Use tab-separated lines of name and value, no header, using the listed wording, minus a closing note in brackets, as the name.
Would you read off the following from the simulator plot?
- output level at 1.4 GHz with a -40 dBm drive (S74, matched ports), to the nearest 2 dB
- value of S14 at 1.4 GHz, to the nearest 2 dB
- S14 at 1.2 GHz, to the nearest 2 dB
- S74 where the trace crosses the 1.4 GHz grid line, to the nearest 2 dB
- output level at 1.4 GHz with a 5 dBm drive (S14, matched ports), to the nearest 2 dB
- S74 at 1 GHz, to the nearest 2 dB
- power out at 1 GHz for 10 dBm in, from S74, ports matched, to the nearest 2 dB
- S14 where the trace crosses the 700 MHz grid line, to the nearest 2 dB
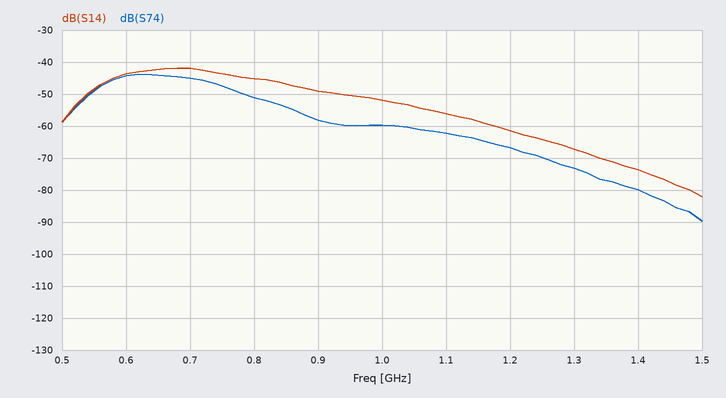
output level at 1.4 GHz with a -40 dBm drive (S74, matched ports), to the nearest 2 dB	-120 dBm
value of S14 at 1.4 GHz, to the nearest 2 dB	-74 dB
S14 at 1.2 GHz, to the nearest 2 dB	-62 dB
S74 where the trace crosses the 1.4 GHz grid line, to the nearest 2 dB	-80 dB
output level at 1.4 GHz with a 5 dBm drive (S14, matched ports), to the nearest 2 dB	-68 dBm
S74 at 1 GHz, to the nearest 2 dB	-60 dB
power out at 1 GHz for 10 dBm in, from S74, ports matched, to the nearest 2 dB	-50 dBm
S14 where the trace crosses the 700 MHz grid line, to the nearest 2 dB	-42 dB
